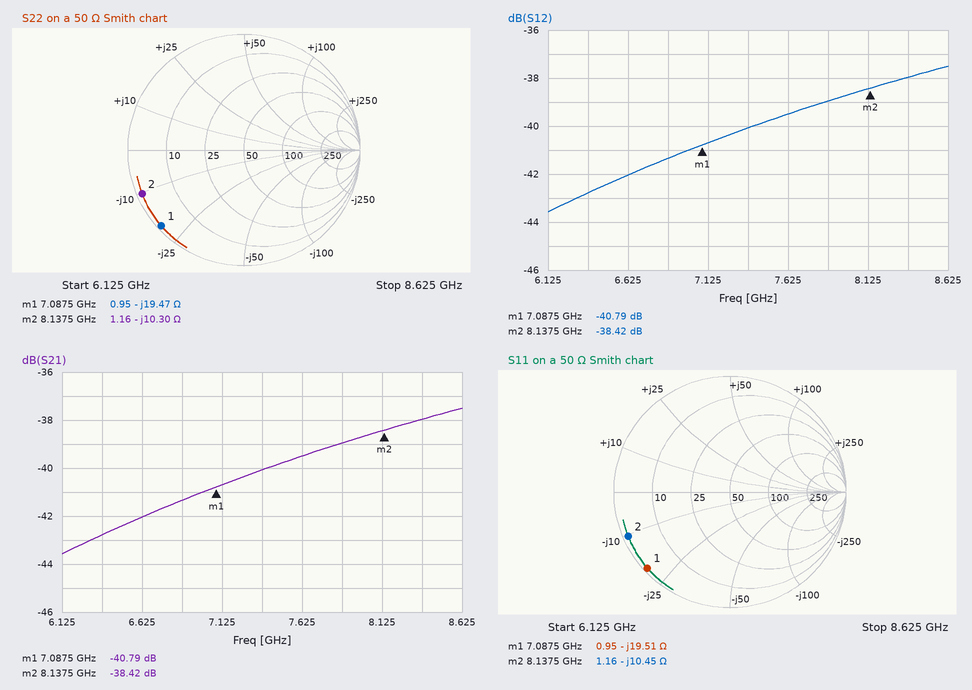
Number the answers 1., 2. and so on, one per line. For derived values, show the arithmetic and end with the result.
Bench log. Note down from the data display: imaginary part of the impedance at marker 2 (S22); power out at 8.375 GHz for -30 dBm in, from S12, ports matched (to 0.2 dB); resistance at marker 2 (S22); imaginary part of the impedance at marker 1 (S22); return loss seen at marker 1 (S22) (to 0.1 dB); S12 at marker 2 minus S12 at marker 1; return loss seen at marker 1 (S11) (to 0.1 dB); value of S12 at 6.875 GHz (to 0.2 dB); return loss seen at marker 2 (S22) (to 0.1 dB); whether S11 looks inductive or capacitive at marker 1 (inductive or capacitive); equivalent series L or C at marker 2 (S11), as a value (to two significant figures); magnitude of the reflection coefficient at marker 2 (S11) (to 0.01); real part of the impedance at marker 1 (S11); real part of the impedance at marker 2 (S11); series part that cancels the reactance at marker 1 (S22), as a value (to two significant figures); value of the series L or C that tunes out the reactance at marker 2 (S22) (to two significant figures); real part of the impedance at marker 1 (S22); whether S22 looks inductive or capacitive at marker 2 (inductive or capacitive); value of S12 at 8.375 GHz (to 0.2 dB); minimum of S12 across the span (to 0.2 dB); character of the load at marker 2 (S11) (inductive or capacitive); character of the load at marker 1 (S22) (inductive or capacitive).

1. -10.30 Ω
2. -30 dBm + (-38.0 dB) = -68.0 dBm
3. 1.16 Ω
4. -19.47 Ω
5. 0.3 dB
6. -38.42 − (-40.79) = 2.37 dB
7. 0.3 dB
8. -41.4 dB
9. 0.4 dB
10. capacitive
11. C = 1/(2π × 8.1375 GHz × 10.45 Ω) ≈ 1.9 pF
12. 0.96
13. 0.95 Ω
14. 1.16 Ω
15. L = 19.47 Ω/(2π × 7.0875 GHz) ≈ 437 pH, so 440 pH to two significant figures
16. L = 10.3 Ω/(2π × 8.1375 GHz) ≈ 201 pH, so 200 pH to two significant figures
17. 0.95 Ω
18. capacitive
19. -38.0 dB
20. -43.6 dB
21. capacitive
22. capacitive
